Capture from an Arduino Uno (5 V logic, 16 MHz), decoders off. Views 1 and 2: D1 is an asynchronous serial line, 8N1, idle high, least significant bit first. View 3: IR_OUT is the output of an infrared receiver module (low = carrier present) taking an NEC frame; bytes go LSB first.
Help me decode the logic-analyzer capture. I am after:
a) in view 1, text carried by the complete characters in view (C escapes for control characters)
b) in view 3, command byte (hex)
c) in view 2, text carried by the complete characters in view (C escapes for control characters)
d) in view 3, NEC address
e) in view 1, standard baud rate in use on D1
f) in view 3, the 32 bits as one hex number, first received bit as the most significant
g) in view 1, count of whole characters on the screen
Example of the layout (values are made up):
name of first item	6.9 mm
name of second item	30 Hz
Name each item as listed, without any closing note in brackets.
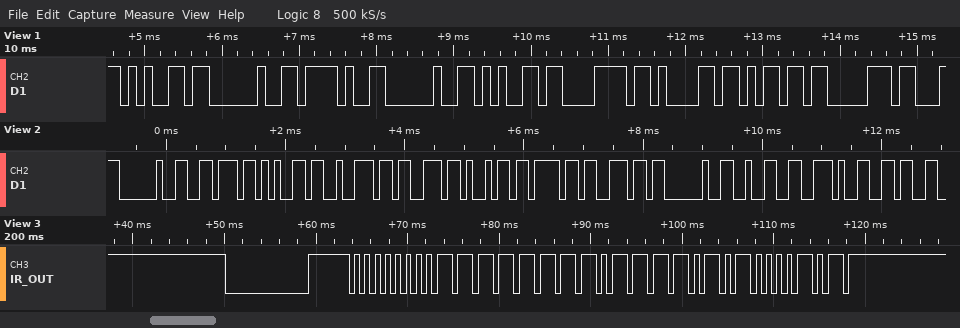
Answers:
in view 1, text carried by the complete characters in view	"e / examp"
in view 3, command byte	0x5E
in view 2, text carried by the complete characters in view	" version 2.6"
in view 3, NEC address	0x00
in view 1, standard baud rate in use on D1	9600 baud
in view 3, the 32 bits as one hex number, first received bit as the most significant	0x00FF7A85
in view 1, count of whole characters on the screen	9
